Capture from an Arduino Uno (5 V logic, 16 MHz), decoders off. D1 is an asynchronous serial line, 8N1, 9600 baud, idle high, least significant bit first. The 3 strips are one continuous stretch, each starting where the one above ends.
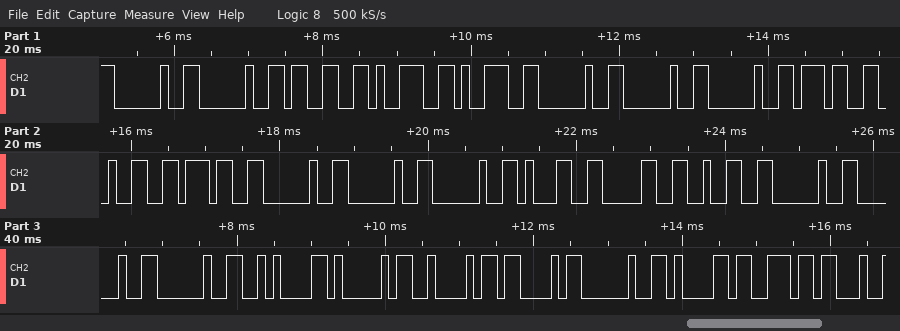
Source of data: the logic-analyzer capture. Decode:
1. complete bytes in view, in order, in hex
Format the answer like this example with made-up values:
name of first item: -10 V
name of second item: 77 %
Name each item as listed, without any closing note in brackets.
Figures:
complete bytes in view, in order, in hex: 20 20 33 39 39 20 20 20 37 32 37 20 20 20 31 30 32 20 20 20 0A 41 42 43 20 61 6E
